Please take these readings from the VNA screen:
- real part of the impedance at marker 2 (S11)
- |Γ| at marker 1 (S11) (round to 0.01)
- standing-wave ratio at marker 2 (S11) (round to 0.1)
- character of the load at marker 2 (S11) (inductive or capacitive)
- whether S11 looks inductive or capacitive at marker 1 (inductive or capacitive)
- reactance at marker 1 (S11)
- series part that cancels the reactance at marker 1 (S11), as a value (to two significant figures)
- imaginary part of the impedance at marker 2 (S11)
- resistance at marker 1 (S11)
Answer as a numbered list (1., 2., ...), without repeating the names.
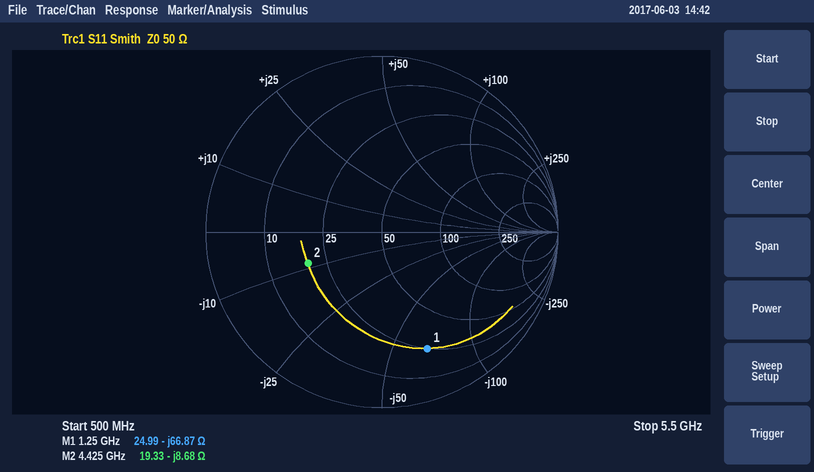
1. 19.33 Ω
2. 0.71
3. 2.7
4. capacitive
5. capacitive
6. -66.87 Ω
7. 8.5 nH
8. -8.68 Ω
9. 24.99 Ω
